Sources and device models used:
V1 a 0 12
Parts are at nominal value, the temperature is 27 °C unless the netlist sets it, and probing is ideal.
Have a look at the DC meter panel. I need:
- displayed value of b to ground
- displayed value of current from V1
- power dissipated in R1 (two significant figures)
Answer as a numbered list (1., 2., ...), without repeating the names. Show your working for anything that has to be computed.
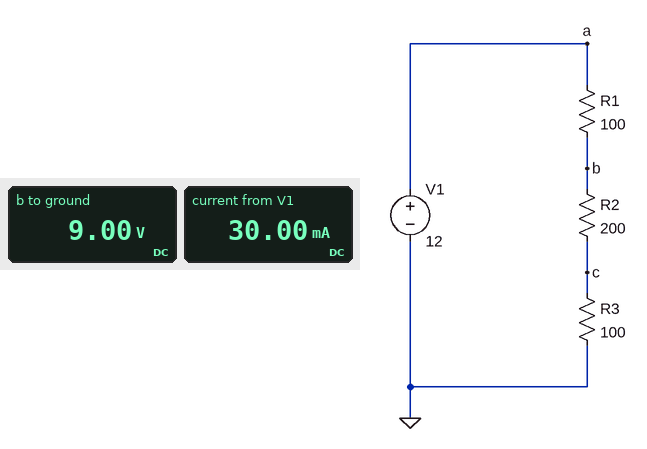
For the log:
1. 9.00 V
2. 30.00 mA
3. (12 V - 9 V)^2 / 100 Ω = 90 mW
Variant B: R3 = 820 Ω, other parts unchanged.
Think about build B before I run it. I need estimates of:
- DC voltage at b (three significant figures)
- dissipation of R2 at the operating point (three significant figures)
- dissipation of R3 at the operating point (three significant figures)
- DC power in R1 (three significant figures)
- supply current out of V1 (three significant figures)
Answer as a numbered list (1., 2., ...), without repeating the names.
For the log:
1. 10.9 V
2. 23.0 mW
3. 94.1 mW
4. 11.5 mW
5. 10.7 mA
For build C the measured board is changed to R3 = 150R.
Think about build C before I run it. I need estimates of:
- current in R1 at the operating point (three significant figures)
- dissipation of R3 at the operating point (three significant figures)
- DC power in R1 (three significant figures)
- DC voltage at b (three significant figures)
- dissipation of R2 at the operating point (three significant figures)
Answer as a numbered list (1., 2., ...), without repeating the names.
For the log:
1. 26.7 mA
2. 107 mW
3. 71.1 mW
4. 9.33 V
5. 142 mW
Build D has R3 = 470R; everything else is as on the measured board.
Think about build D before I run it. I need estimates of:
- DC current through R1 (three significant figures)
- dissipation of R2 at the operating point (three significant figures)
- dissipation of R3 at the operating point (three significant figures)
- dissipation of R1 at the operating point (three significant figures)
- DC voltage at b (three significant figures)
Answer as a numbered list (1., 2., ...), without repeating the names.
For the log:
1. 15.6 mA
2. 48.6 mW
3. 114 mW
4. 24.3 mW
5. 10.4 V
